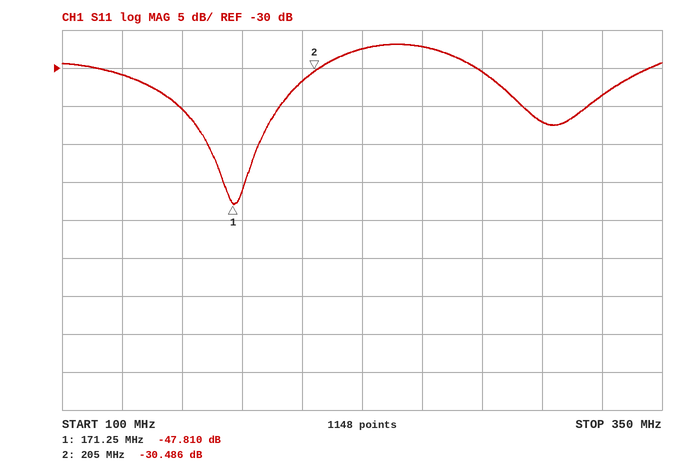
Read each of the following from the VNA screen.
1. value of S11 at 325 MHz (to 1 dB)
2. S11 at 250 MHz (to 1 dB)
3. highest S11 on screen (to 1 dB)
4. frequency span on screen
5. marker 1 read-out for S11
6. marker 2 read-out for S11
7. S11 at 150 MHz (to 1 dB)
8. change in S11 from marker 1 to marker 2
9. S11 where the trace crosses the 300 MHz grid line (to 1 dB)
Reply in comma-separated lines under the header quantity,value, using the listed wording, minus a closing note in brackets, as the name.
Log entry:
quantity,value
value of S11 at 325 MHz,-34 dB
S11 at 250 MHz,-27 dB
highest S11 on screen,-27 dB
frequency span on screen,250 MHz
marker 1 read-out for S11,-47.810 dB
marker 2 read-out for S11,-30.486 dB
S11 at 150 MHz,-35 dB
change in S11 from marker 1 to marker 2,17.324 dB
S11 where the trace crosses the 300 MHz grid line,-37 dB
